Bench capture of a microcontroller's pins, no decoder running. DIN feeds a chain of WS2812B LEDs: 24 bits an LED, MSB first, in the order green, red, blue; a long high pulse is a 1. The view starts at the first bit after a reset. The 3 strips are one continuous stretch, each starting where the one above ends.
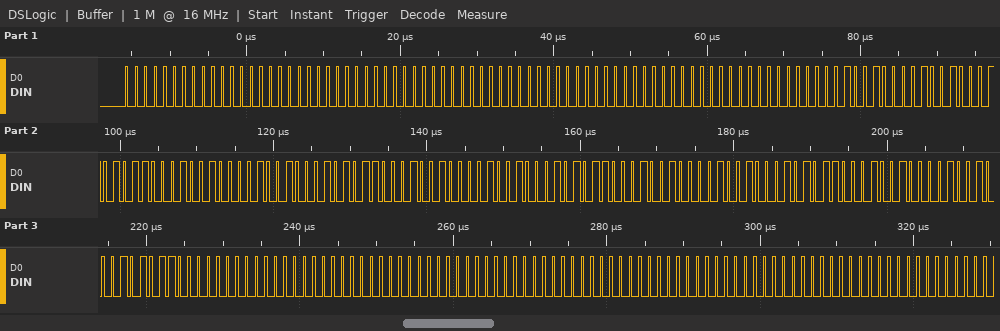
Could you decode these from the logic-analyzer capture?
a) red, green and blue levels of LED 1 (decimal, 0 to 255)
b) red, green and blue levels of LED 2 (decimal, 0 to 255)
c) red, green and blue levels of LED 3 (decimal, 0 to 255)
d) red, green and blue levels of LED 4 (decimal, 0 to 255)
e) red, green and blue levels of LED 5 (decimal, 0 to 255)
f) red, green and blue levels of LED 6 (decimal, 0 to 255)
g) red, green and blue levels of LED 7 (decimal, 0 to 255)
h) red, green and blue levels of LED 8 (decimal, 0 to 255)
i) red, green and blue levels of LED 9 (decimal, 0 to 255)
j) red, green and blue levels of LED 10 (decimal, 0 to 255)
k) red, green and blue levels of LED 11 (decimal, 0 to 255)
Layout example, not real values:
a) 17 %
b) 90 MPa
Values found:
a) 0, 0, 0
b) 0, 0, 0
c) 0, 0, 0
d) 18, 18, 43
e) 18, 18, 43
f) 18, 18, 43
g) 18, 18, 43
h) 18, 18, 43
i) 0, 0, 0
j) 0, 0, 0
k) 0, 0, 0
